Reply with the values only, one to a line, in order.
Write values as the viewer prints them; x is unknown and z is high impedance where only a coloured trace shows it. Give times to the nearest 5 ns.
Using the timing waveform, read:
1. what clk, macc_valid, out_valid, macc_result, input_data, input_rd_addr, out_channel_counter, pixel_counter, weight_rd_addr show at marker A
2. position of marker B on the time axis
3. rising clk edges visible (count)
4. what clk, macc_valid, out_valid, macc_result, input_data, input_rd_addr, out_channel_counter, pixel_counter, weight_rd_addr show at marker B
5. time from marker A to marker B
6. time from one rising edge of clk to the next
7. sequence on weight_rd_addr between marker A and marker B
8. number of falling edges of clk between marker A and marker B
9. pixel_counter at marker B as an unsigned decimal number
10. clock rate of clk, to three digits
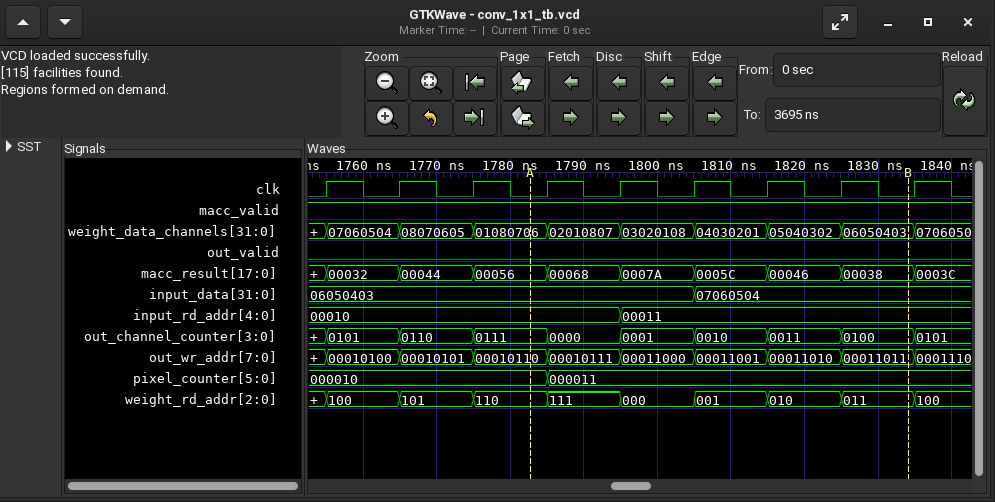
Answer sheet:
clk=0, macc_valid=1, out_valid=0, macc_result=00056, input_data=06050403, input_rd_addr=00010, out_channel_counter=0111, pixel_counter=000010, weight_rd_addr=110
1835 ns
9
clk=0, macc_valid=1, out_valid=0, macc_result=00038, input_data=07060504, input_rd_addr=00011, out_channel_counter=0100, pixel_counter=000011, weight_rd_addr=011
50 ns
10 ns
110, 111, 000, 001, 010, 011
5
3
100 MHz
